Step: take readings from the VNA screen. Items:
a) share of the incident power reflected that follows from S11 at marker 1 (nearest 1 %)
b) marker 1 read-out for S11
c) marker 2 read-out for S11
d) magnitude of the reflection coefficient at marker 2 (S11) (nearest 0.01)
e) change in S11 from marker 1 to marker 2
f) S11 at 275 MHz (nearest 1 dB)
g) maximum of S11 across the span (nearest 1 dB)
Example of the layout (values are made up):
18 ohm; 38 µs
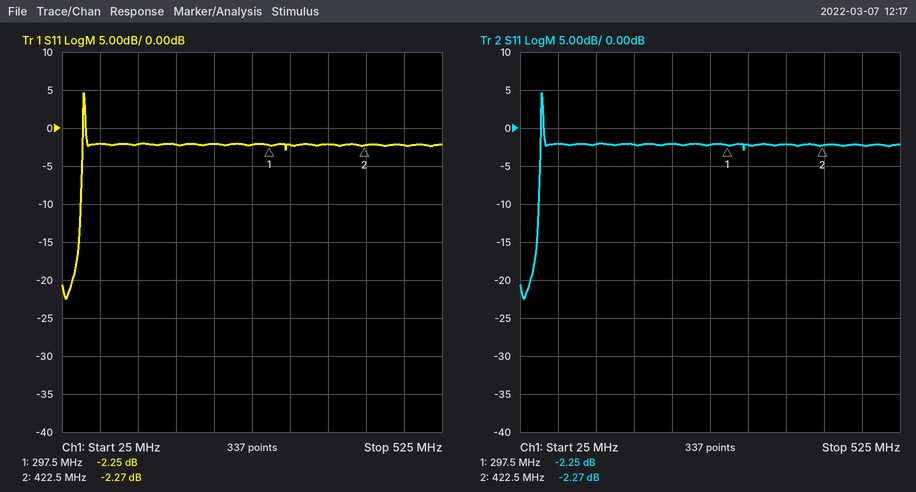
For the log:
60 %; -2.25 dB; -2.27 dB; 0.77; -0.02 dB; -2 dB; 5 dB
